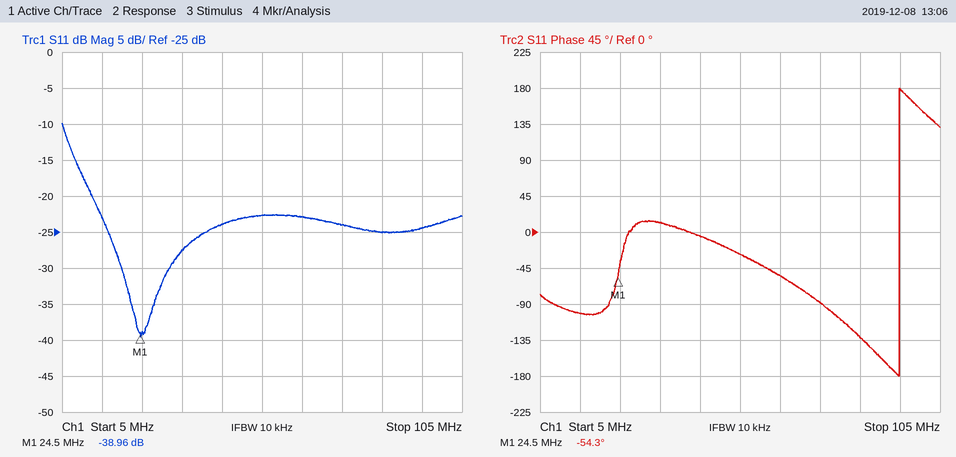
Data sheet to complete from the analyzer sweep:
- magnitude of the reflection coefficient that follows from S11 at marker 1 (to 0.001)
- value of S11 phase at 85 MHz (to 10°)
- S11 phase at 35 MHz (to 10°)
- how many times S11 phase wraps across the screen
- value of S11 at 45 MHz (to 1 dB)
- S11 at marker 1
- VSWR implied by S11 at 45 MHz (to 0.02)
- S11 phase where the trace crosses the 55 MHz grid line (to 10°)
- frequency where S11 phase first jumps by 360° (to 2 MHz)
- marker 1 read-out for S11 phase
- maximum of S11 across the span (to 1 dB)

0.011
-130°
10°
1
-24 dB
-38.96 dB
1.14
-30°
94 MHz
-54.3°
-10 dB
